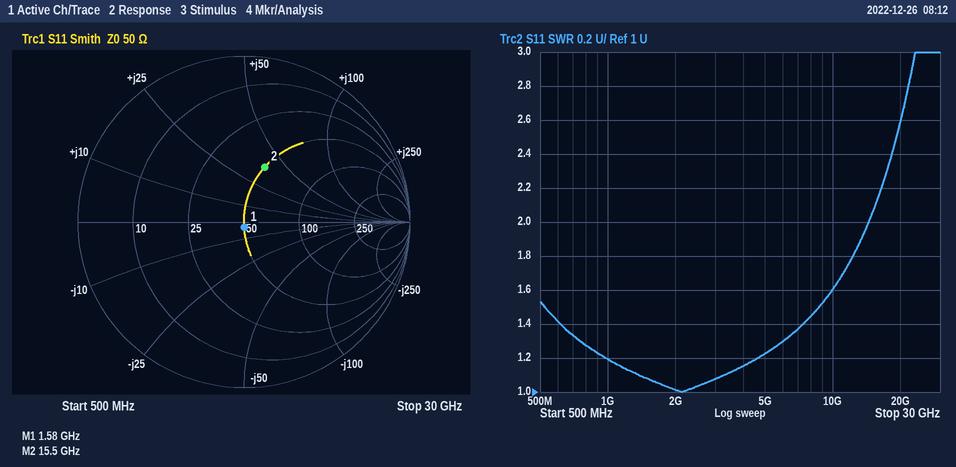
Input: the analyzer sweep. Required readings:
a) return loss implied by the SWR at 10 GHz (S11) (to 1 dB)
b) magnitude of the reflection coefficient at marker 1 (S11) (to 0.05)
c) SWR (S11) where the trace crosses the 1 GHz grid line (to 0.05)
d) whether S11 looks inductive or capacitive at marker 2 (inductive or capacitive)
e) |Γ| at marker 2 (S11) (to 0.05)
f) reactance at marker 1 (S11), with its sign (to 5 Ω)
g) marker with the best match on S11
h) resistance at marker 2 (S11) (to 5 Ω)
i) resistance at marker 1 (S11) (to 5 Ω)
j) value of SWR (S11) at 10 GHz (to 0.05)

13 dB
0.05
1.20
inductive
0.35
-5 Ω
marker 1
50 Ω
50 Ω
1.60
